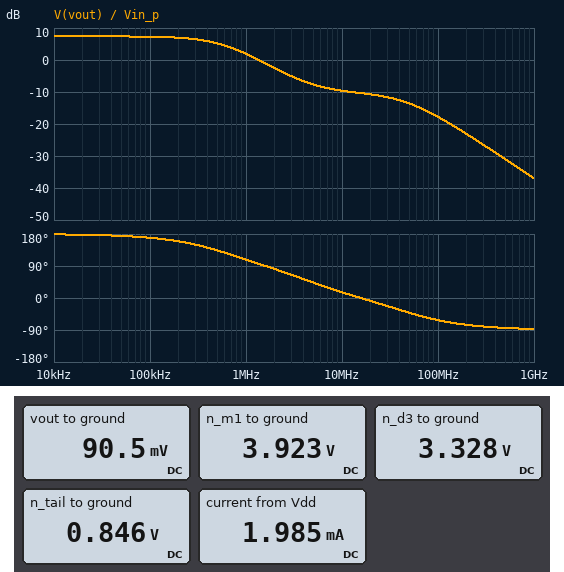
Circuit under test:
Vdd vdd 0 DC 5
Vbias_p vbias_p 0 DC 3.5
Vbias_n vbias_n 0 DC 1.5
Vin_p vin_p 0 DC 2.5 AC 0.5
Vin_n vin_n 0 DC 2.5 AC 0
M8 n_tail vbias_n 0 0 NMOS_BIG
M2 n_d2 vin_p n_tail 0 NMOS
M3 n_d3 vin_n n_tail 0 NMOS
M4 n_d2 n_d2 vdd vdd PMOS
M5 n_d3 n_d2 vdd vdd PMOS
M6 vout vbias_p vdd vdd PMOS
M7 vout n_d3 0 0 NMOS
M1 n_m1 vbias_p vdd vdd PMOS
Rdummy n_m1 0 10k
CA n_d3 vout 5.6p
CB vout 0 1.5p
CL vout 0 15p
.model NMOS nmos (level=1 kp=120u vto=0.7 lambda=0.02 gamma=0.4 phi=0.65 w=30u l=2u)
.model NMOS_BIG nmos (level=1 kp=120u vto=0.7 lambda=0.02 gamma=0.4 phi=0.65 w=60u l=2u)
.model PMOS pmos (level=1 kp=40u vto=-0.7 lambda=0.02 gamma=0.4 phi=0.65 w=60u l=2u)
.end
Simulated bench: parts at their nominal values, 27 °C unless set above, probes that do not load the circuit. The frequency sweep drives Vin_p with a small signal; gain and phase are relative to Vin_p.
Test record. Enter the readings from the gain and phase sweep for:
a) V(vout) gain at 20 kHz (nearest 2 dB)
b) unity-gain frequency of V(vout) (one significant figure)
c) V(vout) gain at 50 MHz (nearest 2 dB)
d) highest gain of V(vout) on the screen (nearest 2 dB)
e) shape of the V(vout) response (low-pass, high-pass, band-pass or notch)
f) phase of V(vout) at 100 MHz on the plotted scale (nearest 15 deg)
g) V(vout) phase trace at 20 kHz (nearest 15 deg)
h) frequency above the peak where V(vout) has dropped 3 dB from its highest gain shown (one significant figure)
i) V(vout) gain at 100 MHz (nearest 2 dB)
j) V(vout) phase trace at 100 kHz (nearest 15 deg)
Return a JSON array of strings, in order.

["8 dB", "1 MHz", "-14 dB", "8 dB", "low-pass", "-60 deg", "180 deg", "600 kHz", "-18 dB", "165 deg"]
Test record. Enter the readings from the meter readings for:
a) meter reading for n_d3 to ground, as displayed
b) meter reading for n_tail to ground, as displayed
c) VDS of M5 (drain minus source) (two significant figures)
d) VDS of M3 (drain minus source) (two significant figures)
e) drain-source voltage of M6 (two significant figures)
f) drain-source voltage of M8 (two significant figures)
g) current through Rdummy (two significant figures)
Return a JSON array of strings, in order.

["3.328 V", "0.846 V", "-1.7 V", "2.5 V", "-4.9 V", "850 mV", "390 µA"]
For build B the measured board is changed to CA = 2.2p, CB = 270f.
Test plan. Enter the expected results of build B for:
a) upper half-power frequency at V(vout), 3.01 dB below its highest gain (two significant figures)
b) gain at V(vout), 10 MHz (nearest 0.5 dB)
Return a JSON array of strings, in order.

["1.6 MHz", "-6.5 dB"]
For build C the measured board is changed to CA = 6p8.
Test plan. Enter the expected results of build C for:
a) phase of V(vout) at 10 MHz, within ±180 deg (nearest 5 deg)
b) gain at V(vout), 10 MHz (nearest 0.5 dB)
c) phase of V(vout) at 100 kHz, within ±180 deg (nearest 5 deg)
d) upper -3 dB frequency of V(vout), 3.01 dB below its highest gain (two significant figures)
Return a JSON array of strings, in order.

["10 deg", "-10.0 dB", "165 deg", "510 kHz"]
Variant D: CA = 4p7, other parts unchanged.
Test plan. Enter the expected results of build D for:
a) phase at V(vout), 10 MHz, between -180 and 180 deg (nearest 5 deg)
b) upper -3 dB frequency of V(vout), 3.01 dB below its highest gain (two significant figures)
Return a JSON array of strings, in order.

["20 deg", "740 kHz"]
